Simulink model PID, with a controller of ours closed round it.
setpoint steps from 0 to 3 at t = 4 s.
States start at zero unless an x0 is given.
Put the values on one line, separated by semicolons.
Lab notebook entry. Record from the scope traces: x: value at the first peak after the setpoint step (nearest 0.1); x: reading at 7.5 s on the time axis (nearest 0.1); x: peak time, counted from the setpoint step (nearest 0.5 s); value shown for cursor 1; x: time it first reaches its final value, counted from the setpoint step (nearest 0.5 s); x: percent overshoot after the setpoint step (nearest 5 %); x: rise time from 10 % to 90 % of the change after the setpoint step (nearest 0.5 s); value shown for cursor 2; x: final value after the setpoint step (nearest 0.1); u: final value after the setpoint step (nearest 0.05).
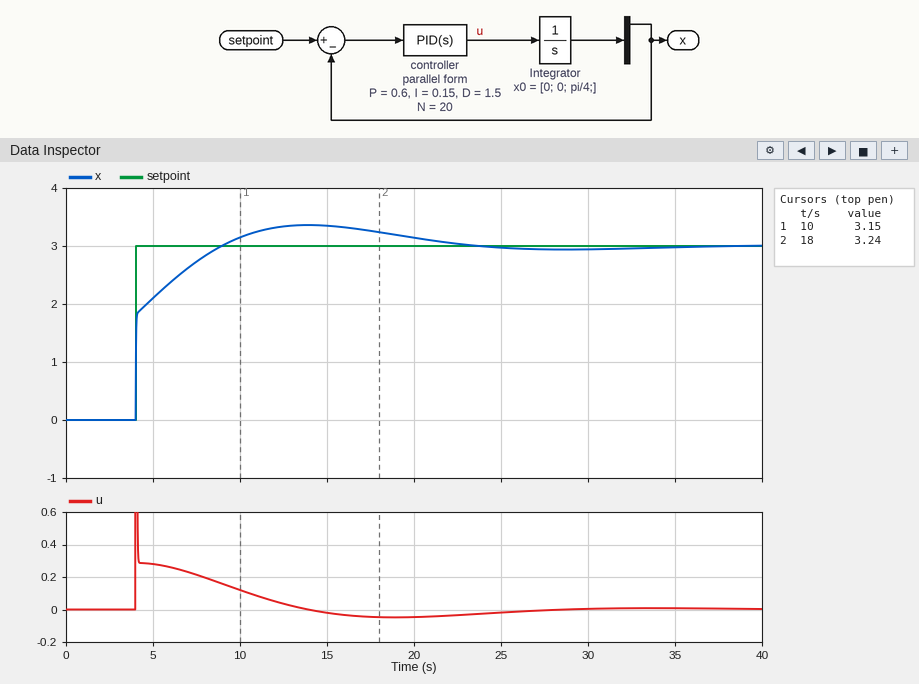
3.4; 2.7; 10.0 s; 3.15; 5.0 s; 10 %; 3.5 s; 3.24; 3.0; 0.00
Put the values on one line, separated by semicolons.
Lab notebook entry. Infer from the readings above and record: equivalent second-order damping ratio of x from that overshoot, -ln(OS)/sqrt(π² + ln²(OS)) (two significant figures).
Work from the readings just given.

0.59
